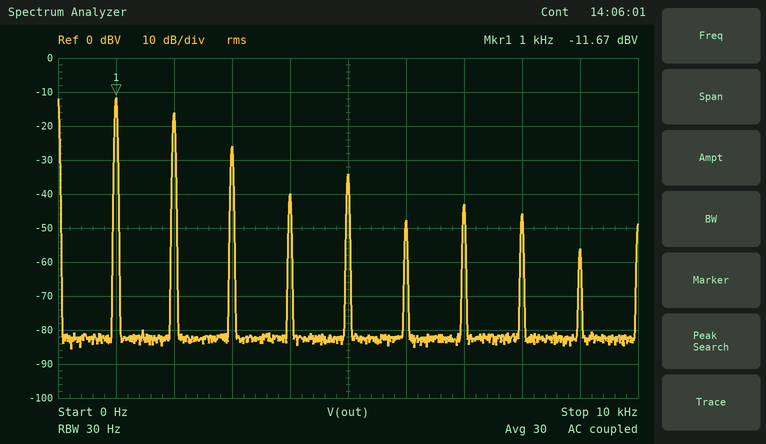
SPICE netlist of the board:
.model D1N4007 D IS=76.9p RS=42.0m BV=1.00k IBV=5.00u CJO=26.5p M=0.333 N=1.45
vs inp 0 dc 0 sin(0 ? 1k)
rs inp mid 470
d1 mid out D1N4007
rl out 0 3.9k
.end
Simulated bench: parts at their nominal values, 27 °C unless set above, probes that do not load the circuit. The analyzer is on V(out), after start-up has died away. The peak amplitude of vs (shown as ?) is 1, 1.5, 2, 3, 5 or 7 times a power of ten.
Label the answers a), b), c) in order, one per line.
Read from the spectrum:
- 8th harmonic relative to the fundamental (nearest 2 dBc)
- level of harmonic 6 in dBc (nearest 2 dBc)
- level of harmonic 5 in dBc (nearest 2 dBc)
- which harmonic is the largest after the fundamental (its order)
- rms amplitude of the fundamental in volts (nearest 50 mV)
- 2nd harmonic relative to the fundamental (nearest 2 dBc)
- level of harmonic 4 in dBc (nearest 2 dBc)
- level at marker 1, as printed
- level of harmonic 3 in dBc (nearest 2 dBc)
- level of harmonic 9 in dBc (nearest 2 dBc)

a) -34 dBc
b) -36 dBc
c) -22 dBc
d) 2
e) 250 mV
f) -4 dBc
g) -28 dBc
h) -11.67 dBV
i) -14 dBc
j) -44 dBc
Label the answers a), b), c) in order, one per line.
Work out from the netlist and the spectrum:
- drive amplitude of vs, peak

a) 1.5 V
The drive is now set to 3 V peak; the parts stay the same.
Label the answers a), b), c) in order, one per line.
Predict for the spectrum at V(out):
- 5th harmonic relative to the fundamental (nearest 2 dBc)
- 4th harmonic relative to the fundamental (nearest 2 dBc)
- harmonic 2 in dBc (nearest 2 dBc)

a) -26 dBc
b) -22 dBc
c) -6 dBc
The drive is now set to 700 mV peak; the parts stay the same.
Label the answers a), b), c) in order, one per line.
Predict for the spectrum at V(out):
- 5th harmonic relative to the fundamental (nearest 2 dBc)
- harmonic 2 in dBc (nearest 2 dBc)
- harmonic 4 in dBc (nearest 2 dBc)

a) -36 dBc
b) -2 dBc
c) -14 dBc
